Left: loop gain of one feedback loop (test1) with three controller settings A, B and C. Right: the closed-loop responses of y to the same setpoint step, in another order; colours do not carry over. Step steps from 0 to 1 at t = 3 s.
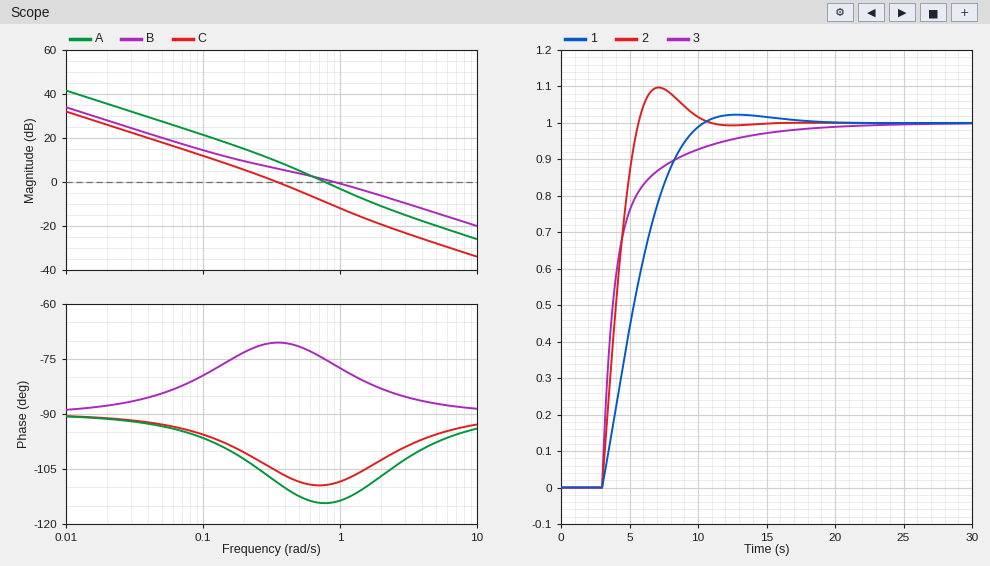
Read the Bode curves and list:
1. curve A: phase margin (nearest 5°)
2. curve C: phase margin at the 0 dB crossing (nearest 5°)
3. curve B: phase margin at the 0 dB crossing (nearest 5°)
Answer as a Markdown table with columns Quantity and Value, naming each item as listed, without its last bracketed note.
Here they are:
| Quantity | Value |
|---|---|
| curve A: phase margin | 65° |
| curve C: phase margin at the 0 dB crossing | 75° |
| curve B: phase margin at the 0 dB crossing | 105° |
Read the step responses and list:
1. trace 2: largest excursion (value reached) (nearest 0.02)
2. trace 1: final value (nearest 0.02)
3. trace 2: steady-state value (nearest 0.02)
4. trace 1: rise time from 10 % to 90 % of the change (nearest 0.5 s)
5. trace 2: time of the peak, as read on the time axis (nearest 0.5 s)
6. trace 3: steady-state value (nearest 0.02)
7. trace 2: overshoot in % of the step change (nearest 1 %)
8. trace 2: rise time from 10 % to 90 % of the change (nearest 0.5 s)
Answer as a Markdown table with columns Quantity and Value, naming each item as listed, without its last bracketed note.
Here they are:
| Quantity | Value |
|---|---|
| trace 2: largest excursion (value reached) | 1.10 |
| trace 1: final value | 1.00 |
| trace 2: steady-state value | 1.00 |
| trace 1: rise time from 10 % to 90 % of the change | 5.0 s |
| trace 2: time of the peak, as read on the time axis | 7.0 s |
| trace 3: steady-state value | 1.00 |
| trace 2: overshoot in % of the step change | 10 % |
| trace 2: rise time from 10 % to 90 % of the change | 2.0 s |
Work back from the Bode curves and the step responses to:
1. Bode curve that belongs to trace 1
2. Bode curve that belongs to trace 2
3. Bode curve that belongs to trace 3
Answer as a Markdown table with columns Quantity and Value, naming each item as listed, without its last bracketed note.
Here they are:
| Quantity | Value |
|---|---|
| Bode curve that belongs to trace 1 | C |
| Bode curve that belongs to trace 2 | A |
| Bode curve that belongs to trace 3 | B |
